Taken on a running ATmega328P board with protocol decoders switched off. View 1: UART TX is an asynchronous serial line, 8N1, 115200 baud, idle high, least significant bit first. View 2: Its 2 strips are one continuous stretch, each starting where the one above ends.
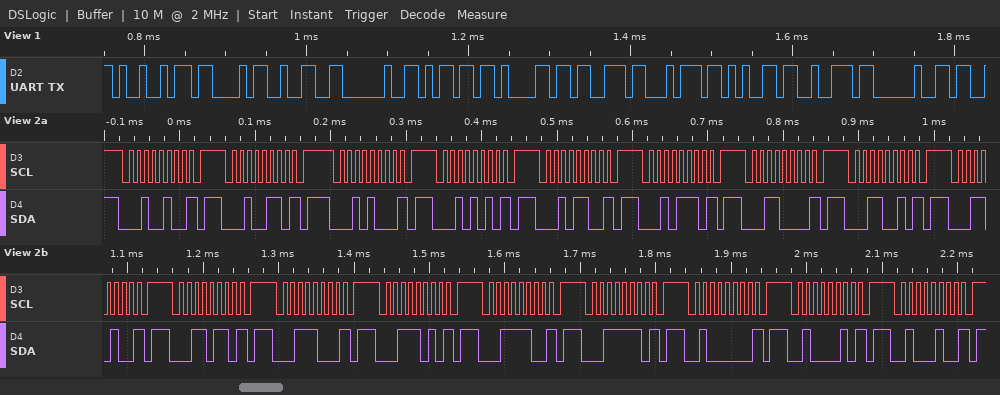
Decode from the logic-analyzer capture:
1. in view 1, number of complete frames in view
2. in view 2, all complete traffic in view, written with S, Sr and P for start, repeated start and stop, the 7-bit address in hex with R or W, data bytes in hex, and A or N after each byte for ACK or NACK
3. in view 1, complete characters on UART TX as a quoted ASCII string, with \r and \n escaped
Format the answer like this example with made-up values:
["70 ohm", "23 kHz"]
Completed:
["11", "S 12W N P S 13W N P S 14W N P S 15W N P S 16W N P S 17W N P S 18W N P S 19W N P S 1AW N P S 1BW N P S 1CW N P S 1DW N P S 1EW N P S 1FW N P S 20W N P S 21W N P S 22W N P", "\"IC2 master \""]
